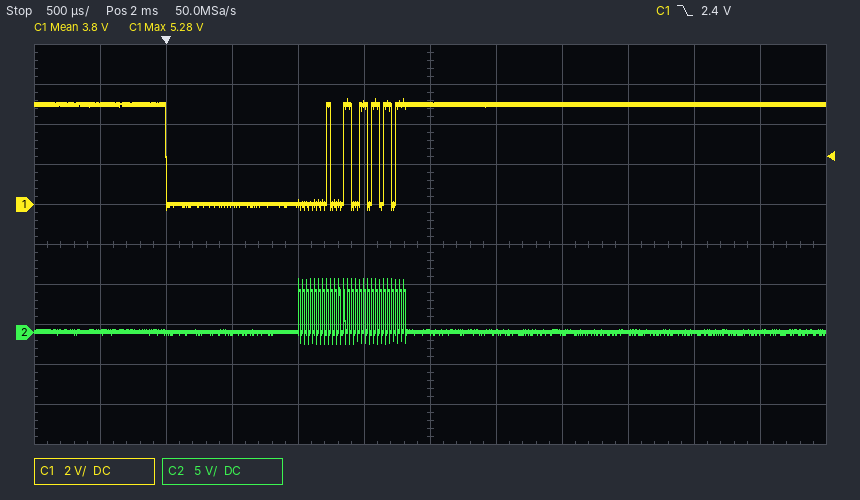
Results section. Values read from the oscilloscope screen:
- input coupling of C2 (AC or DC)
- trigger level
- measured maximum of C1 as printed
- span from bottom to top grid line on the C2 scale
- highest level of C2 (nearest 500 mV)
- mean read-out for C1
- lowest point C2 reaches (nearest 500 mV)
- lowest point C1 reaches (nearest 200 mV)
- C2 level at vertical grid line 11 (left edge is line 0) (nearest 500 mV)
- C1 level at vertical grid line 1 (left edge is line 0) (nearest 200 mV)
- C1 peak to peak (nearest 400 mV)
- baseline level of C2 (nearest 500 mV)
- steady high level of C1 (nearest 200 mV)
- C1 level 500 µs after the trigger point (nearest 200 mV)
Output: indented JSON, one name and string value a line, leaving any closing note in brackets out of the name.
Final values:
{
  "input coupling of C2": "DC",
  "trigger level": "2.4 V",
  "measured maximum of C1 as printed": "5.28 V",
  "span from bottom to top grid line on the C2 scale": "50 V",
  "highest level of C2": "7.0 V",
  "mean read-out for C1": "3.8 V",
  "lowest point C2 reaches": "-1.5 V",
  "lowest point C1 reaches": "-200 mV",
  "C2 level at vertical grid line 11 (left edge is line 0)": "0.0 V",
  "C1 level at vertical grid line 1 (left edge is line 0)": "5.0 V",
  "C1 peak to peak": "5.6 V",
  "baseline level of C2": "0.0 V",
  "steady high level of C1": "5.0 V",
  "C1 level 500 µs after the trigger point": "0.0 V"
}
